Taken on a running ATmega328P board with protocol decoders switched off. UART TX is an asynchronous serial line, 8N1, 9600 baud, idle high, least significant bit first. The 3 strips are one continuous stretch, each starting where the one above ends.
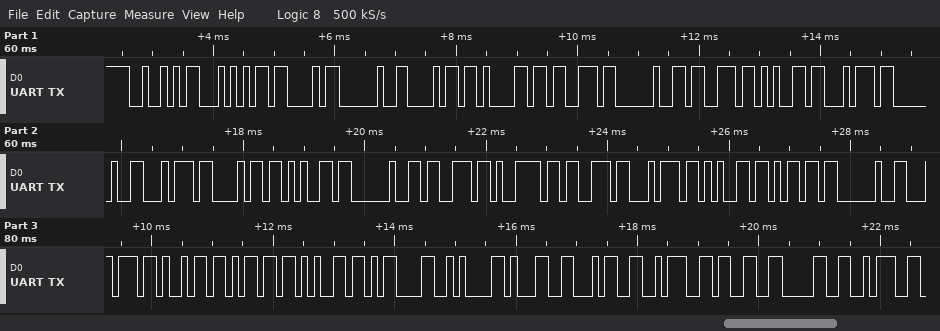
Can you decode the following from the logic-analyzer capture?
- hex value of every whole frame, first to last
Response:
0x52 0x54 0x43 0x20 0x68 0x61 0x73 0x20 0x73 0x65 0x74 0x20 0x74 0x68 0x65 0x20 0x73 0x79 0x73 0x74 0x65 0x6D 0x20 0x74 0x69 0x6D 0x65 0x0D 0x0A 0x31 0x34 0x3A 0x33 0x30 0x3A
